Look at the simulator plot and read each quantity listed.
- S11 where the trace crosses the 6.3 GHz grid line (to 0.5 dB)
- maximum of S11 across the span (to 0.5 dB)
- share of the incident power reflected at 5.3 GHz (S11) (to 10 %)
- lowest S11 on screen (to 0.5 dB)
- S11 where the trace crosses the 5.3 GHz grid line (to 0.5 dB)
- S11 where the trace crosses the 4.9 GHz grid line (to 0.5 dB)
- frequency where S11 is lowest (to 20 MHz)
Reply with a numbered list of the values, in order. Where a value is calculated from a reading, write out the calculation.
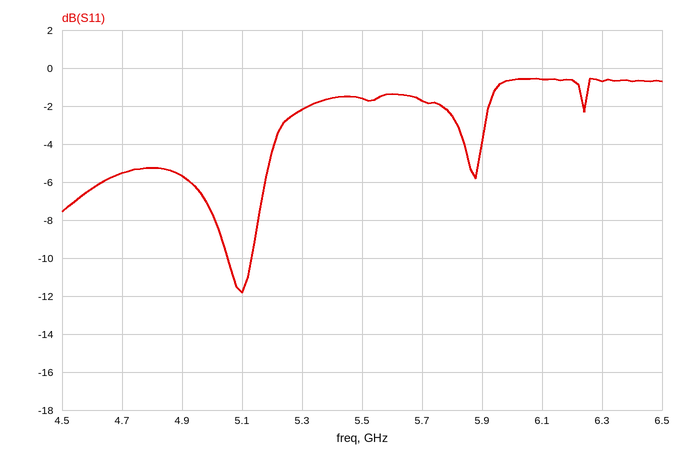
1. -0.5 dB
2. -0.5 dB
3. 10^(-2/10) ≈ 63.1 %, so 60 % to the nearest 10 %
4. -12.0 dB
5. -2.0 dB
6. -5.5 dB
7. 5.10 GHz
